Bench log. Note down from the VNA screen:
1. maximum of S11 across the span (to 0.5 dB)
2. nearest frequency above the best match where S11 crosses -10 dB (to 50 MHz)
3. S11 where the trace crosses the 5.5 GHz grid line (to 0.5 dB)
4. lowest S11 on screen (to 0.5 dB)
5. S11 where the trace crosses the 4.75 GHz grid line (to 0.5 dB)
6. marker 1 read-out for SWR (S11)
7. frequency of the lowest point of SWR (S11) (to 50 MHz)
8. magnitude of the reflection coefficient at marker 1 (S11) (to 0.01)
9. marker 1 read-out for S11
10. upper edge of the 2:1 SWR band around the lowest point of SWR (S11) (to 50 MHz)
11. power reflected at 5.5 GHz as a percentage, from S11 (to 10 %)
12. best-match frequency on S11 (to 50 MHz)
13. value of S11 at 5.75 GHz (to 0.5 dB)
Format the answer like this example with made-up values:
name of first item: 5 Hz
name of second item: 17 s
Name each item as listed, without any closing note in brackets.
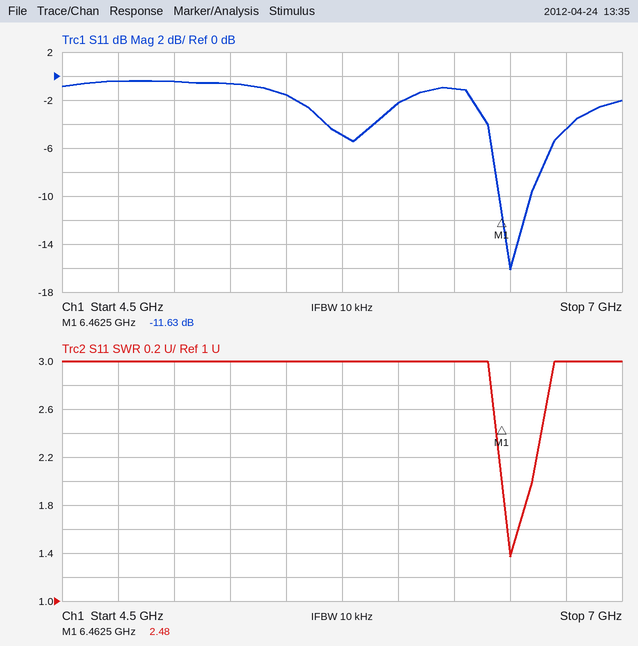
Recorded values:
maximum of S11 across the span: -0.5 dB
nearest frequency above the best match where S11 crosses -10 dB: 6.60 GHz
S11 where the trace crosses the 5.5 GHz grid line: -1.5 dB
lowest S11 on screen: -16.0 dB
S11 where the trace crosses the 4.75 GHz grid line: -0.5 dB
marker 1 read-out for SWR: 2.48
frequency of the lowest point of SWR (S11): 6.50 GHz
magnitude of the reflection coefficient at marker 1 (S11): 0.26
marker 1 read-out for S11: -11.63 dB
upper edge of the 2:1 SWR band around the lowest point of SWR (S11): 6.60 GHz
power reflected at 5.5 GHz as a percentage, from S11: 70 %
best-match frequency on S11: 6.50 GHz
value of S11 at 5.75 GHz: -5.0 dB
